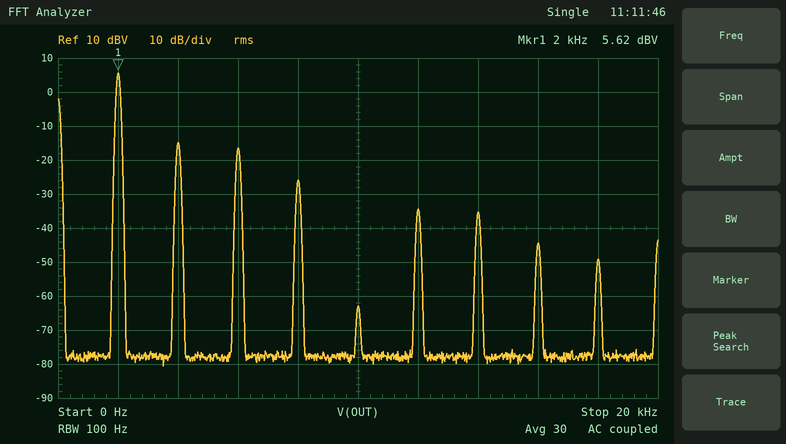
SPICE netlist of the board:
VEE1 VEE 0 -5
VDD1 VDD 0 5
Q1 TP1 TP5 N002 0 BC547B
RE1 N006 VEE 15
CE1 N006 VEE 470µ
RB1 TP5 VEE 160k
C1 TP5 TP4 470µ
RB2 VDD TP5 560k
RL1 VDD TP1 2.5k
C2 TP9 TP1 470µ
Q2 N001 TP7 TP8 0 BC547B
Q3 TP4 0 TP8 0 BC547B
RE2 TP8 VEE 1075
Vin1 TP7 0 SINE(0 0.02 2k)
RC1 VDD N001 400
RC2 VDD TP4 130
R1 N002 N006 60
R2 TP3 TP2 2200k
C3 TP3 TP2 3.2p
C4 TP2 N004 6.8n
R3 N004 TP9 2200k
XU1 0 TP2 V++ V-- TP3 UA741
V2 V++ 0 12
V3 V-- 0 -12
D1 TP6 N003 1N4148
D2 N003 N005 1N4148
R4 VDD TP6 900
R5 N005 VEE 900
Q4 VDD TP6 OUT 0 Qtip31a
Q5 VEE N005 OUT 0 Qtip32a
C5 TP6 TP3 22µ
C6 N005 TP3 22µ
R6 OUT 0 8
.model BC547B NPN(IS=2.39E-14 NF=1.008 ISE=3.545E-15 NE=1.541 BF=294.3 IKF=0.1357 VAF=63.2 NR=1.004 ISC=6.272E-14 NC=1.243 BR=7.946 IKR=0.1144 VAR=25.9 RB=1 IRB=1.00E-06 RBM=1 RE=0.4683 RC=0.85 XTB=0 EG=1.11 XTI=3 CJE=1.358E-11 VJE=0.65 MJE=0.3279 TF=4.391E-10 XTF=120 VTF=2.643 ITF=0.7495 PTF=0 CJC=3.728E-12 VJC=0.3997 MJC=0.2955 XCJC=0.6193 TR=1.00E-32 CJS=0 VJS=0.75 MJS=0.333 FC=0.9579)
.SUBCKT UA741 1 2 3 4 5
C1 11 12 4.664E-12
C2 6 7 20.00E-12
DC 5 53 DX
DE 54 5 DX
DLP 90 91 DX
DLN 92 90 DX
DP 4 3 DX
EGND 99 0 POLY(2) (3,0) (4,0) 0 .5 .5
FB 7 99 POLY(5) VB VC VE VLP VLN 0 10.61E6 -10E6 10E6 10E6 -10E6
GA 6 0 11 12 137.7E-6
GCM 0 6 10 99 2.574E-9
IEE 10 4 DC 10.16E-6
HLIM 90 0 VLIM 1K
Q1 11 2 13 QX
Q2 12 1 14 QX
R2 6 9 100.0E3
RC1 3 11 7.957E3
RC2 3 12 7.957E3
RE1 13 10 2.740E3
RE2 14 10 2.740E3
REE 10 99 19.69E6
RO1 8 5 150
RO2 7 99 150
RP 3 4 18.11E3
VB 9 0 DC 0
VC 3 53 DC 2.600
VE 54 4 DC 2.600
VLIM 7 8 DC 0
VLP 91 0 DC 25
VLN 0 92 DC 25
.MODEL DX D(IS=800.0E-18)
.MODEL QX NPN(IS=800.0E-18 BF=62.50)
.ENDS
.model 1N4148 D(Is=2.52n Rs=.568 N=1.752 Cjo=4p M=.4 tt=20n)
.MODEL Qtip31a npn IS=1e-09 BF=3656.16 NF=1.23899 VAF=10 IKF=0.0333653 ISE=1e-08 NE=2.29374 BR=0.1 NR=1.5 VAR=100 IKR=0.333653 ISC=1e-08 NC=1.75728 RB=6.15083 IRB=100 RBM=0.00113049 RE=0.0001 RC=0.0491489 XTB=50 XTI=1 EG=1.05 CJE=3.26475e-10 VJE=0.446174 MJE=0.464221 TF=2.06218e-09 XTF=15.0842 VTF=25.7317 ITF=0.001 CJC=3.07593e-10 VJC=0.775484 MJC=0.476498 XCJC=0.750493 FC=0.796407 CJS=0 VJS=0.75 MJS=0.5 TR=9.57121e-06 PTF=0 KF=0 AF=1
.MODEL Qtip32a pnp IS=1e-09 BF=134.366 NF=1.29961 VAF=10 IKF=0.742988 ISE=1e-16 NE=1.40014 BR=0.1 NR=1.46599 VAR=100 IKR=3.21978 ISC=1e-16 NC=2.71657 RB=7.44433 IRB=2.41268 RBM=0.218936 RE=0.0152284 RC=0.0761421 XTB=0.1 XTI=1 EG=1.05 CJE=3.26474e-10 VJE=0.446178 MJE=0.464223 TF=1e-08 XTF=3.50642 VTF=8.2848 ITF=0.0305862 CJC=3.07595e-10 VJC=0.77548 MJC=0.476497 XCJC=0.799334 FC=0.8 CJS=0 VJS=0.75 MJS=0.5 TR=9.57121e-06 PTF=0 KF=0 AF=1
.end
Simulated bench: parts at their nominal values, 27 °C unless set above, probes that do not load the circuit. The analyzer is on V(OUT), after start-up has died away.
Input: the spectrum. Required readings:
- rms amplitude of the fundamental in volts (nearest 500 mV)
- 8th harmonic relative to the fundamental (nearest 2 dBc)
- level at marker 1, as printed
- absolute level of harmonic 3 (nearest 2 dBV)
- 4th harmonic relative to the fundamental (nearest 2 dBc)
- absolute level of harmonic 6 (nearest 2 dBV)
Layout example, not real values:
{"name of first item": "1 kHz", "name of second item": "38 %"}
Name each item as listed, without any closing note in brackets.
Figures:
{"rms amplitude of the fundamental in volts": "2.0 V", "8th harmonic relative to the fundamental": "-50 dBc", "level at marker 1, as printed": "5.62 dBV", "absolute level of harmonic 3": "-16 dBV", "4th harmonic relative to the fundamental": "-32 dBc", "absolute level of harmonic 6": "-34 dBV"}
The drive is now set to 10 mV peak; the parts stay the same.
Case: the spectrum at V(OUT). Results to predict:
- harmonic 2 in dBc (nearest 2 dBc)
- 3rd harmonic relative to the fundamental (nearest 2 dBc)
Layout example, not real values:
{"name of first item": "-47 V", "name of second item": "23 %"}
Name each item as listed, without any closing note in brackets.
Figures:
{"harmonic 2 in dBc": "-44 dBc", "3rd harmonic relative to the fundamental": "-50 dBc"}
